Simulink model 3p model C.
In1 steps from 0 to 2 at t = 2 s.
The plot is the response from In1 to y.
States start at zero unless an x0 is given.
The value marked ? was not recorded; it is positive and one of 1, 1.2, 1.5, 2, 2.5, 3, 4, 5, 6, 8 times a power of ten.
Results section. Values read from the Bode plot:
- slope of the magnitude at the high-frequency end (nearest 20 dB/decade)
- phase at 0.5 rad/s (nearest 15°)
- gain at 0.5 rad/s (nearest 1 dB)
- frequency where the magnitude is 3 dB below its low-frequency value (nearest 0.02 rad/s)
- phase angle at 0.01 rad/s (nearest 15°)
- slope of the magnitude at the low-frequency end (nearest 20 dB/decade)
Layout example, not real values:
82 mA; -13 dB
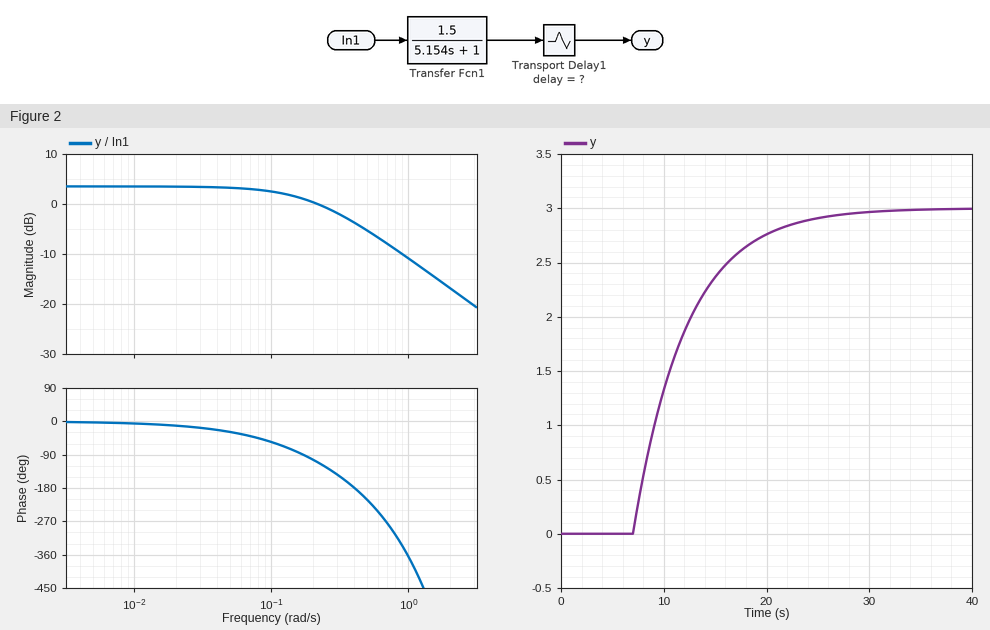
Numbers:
-20 dB/decade; -210°; -5 dB; 0.20 rad/s; 0°; 0 dB/decade
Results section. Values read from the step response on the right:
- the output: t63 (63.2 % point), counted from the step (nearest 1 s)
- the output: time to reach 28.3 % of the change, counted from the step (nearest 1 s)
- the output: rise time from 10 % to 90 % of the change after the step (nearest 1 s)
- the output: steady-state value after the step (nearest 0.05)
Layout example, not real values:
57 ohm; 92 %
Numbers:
10 s; 7 s; 11 s; 3.00
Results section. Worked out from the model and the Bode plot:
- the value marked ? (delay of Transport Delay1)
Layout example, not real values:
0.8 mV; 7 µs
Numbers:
5
